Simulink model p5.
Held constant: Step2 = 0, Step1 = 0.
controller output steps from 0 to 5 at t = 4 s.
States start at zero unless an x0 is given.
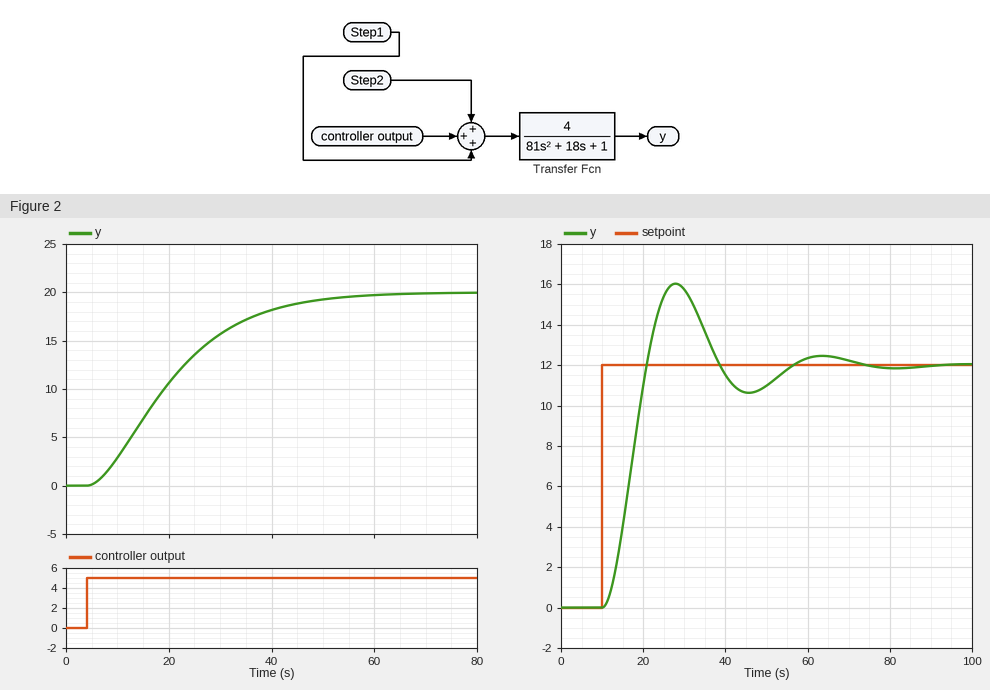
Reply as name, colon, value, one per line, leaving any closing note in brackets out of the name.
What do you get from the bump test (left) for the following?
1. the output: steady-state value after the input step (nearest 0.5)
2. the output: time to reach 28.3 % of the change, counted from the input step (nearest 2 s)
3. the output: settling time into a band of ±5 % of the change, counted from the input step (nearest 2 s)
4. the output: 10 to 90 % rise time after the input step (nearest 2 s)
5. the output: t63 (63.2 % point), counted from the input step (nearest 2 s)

the output: steady-state value after the input step: 20.0
the output: time to reach 28.3 % of the change, counted from the input step: 10 s
the output: settling time into a band of ±5 % of the change, counted from the input step: 42 s
the output: 10 to 90 % rise time after the input step: 30 s
the output: t63 (63.2 % point), counted from the input step: 20 s
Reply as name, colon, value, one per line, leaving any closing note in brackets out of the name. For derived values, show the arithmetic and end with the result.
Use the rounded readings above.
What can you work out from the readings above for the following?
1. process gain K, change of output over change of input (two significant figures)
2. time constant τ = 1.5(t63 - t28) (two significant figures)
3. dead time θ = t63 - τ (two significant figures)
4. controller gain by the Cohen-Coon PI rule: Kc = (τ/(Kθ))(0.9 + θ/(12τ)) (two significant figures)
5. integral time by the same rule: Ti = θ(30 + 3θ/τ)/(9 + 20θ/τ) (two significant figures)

process gain K, change of output over change of input: (20 - 0) / 5 = 4.0
time constant τ = 1.5(t63 - t28): 1.5 × (20 - 10) = 15 s
dead time θ = t63 - τ: 20 - 15 = 5.0 s
controller gain by the Cohen-Coon PI rule: Kc = (τ/(Kθ))(0.9 + θ/(12τ)): 15 / (4 × 5) × (0.9 + 5 / (12 × 15)) = 0.70
integral time by the same rule: Ti = θ(30 + 3θ/τ)/(9 + 20θ/τ): 5 × (30 + 3 × 5 / 15) / (9 + 20 × 5 / 15) = 9.9 s
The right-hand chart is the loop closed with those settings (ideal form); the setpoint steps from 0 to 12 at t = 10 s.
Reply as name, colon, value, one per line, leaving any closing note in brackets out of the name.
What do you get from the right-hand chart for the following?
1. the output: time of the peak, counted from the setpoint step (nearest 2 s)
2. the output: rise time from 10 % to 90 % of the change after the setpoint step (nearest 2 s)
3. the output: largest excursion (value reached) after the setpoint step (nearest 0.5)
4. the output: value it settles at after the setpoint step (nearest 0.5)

the output: time of the peak, counted from the setpoint step: 18 s
the output: rise time from 10 % to 90 % of the change after the setpoint step: 8 s
the output: largest excursion (value reached) after the setpoint step: 16.0
the output: value it settles at after the setpoint step: 12.0
